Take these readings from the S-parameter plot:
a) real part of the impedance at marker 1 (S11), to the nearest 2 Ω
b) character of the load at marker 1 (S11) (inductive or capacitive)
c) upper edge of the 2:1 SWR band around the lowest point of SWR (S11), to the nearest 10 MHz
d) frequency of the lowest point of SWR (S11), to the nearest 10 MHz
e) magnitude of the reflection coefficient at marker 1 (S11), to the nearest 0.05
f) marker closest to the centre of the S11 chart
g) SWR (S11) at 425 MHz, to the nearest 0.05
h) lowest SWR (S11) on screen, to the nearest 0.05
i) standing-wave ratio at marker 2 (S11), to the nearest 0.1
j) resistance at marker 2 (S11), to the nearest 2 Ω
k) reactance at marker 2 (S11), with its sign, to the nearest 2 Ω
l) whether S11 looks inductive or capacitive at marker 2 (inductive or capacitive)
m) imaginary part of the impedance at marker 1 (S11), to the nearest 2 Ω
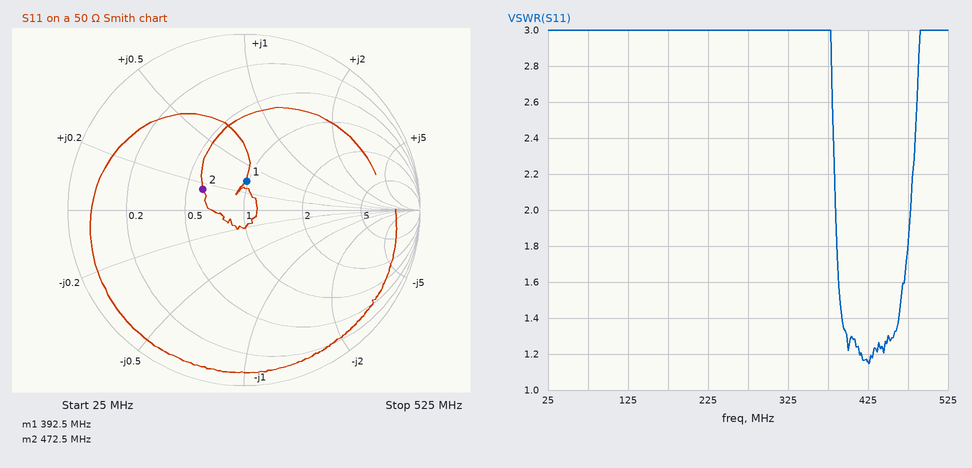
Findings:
48 Ω
inductive
480 MHz
430 MHz
0.15
marker 1
1.15
1.15
1.7
30 Ω
+8 Ω
inductive
+16 Ω
